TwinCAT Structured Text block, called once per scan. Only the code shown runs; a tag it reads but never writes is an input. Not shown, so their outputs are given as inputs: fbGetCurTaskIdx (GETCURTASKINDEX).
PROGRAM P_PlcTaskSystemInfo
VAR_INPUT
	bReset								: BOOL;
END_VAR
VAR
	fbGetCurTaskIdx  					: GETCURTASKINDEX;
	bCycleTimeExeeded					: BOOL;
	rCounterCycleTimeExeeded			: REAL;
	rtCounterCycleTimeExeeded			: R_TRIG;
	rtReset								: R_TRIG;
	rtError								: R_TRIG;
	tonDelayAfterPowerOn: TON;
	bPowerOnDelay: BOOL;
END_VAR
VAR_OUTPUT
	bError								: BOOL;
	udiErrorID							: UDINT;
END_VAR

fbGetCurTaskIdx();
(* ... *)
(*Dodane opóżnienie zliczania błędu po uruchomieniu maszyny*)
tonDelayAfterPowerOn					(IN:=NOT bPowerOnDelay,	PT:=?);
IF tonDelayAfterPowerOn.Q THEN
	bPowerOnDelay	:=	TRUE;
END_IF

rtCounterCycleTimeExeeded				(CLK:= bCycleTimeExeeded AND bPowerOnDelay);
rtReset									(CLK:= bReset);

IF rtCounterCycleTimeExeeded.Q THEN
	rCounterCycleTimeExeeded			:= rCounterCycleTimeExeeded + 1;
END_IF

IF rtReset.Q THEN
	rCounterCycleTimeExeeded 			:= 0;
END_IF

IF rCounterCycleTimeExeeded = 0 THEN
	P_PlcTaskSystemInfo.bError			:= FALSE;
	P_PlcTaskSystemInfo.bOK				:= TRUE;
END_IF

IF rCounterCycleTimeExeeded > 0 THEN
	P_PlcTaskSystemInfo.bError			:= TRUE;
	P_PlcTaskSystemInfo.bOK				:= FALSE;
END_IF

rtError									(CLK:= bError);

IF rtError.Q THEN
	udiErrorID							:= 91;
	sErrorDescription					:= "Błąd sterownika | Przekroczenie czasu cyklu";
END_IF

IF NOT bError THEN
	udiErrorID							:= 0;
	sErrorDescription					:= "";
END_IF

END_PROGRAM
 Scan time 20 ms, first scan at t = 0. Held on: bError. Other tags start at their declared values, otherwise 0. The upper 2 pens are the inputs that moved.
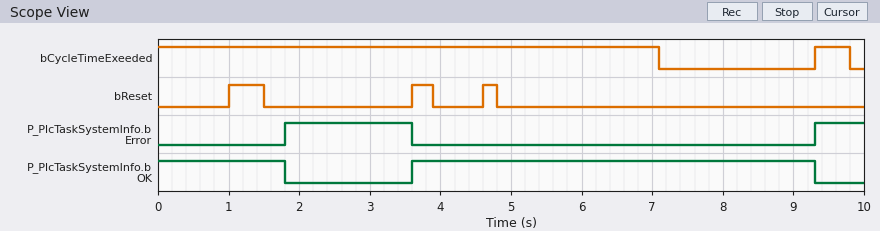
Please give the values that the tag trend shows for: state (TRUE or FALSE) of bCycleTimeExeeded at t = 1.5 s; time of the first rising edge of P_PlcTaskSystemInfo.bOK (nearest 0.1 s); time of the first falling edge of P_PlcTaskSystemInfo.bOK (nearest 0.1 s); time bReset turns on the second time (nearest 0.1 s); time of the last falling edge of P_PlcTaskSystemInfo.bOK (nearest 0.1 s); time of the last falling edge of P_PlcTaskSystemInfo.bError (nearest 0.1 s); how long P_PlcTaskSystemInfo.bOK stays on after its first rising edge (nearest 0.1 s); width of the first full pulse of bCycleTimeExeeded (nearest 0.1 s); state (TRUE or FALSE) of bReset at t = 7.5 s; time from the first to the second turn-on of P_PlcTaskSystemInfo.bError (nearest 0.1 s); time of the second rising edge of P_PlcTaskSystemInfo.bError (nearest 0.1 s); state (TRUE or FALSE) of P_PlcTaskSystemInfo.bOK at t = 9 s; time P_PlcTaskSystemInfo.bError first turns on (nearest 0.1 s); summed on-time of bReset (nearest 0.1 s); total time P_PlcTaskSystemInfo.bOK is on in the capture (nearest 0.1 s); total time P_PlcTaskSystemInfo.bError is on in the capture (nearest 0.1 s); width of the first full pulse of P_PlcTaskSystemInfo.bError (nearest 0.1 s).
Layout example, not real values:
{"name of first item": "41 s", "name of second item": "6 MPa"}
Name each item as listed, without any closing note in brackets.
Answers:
{"state (TRUE or FALSE) of bCycleTimeExeeded at t = 1.5 s": "TRUE", "time of the first rising edge of P_PlcTaskSystemInfo.bOK": "3.6 s", "time of the first falling edge of P_PlcTaskSystemInfo.bOK": "1.8 s", "time bReset turns on the second time": "3.6 s", "time of the last falling edge of P_PlcTaskSystemInfo.bOK": "9.3 s", "time of the last falling edge of P_PlcTaskSystemInfo.bError": "3.6 s", "how long P_PlcTaskSystemInfo.bOK stays on after its first rising edge": "5.7 s", "width of the first full pulse of bCycleTimeExeeded": "0.5 s", "state (TRUE or FALSE) of bReset at t = 7.5 s": "FALSE", "time from the first to the second turn-on of P_PlcTaskSystemInfo.bError": "7.5 s", "time of the second rising edge of P_PlcTaskSystemInfo.bError": "9.3 s", "state (TRUE or FALSE) of P_PlcTaskSystemInfo.bOK at t = 9 s": "TRUE", "time P_PlcTaskSystemInfo.bError first turns on": "1.8 s", "summed on-time of bReset": "1.0 s", "total time P_PlcTaskSystemInfo.bOK is on in the capture": "7.5 s", "total time P_PlcTaskSystemInfo.bError is on in the capture": "2.5 s", "width of the first full pulse of P_PlcTaskSystemInfo.bError": "1.8 s"}
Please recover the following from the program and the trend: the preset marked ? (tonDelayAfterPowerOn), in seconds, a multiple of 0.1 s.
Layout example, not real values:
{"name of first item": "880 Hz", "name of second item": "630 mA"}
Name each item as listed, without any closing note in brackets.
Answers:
{"the preset marked ? (tonDelayAfterPowerOn), in seconds, a multiple of 0.1 s": "1.8 s"}
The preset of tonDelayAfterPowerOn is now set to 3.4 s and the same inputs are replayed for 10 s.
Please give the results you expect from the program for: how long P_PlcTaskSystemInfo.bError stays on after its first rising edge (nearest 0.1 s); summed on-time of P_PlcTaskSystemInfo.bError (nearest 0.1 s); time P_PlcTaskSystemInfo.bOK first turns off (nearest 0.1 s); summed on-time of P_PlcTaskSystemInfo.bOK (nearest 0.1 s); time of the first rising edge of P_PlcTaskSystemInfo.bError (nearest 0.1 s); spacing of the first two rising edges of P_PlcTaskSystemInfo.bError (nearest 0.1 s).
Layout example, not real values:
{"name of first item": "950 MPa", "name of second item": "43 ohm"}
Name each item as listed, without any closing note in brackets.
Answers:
{"how long P_PlcTaskSystemInfo.bError stays on after its first rising edge": "0.2 s", "summed on-time of P_PlcTaskSystemInfo.bError": "0.9 s", "time P_PlcTaskSystemInfo.bOK first turns off": "3.4 s", "summed on-time of P_PlcTaskSystemInfo.bOK": "9.1 s", "time of the first rising edge of P_PlcTaskSystemInfo.bError": "3.4 s", "spacing of the first two rising edges of P_PlcTaskSystemInfo.bError": "5.9 s"}
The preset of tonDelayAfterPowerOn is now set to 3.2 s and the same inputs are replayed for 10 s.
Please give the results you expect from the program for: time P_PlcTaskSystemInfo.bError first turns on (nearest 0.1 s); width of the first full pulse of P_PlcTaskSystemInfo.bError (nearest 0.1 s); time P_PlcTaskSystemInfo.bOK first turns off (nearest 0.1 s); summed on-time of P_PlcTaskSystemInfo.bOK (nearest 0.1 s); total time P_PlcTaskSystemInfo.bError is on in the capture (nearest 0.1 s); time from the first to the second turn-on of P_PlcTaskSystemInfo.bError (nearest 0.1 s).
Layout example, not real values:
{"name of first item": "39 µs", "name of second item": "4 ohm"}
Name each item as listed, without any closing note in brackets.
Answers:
{"time P_PlcTaskSystemInfo.bError first turns on": "3.2 s", "width of the first full pulse of P_PlcTaskSystemInfo.bError": "0.4 s", "time P_PlcTaskSystemInfo.bOK first turns off": "3.2 s", "summed on-time of P_PlcTaskSystemInfo.bOK": "8.9 s", "total time P_PlcTaskSystemInfo.bError is on in the capture": "1.1 s", "time from the first to the second turn-on of P_PlcTaskSystemInfo.bError": "6.1 s"}
